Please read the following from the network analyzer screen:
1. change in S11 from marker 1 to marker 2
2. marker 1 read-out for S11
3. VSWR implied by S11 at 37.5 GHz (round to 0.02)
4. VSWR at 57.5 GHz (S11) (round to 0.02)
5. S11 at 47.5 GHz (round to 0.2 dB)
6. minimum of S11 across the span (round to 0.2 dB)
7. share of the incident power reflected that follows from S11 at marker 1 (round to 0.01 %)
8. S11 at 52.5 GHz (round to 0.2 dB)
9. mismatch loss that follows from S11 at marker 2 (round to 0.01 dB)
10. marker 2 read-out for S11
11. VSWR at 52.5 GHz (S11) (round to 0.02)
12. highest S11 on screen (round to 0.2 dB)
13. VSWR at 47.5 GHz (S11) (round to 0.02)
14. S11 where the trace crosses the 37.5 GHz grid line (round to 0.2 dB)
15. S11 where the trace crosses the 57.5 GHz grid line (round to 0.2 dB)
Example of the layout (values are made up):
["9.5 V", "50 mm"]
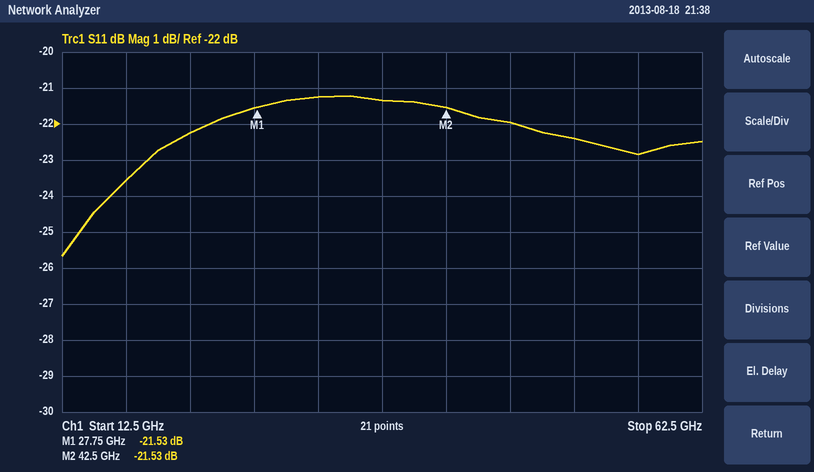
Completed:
["0.00 dB", "-21.53 dB", "1.18", "1.16", "-22.0 dB", "-25.6 dB", "0.70 %", "-22.4 dB", "0.03 dB", "-21.53 dB", "1.16", "-21.2 dB", "1.18", "-21.4 dB", "-22.8 dB"]
